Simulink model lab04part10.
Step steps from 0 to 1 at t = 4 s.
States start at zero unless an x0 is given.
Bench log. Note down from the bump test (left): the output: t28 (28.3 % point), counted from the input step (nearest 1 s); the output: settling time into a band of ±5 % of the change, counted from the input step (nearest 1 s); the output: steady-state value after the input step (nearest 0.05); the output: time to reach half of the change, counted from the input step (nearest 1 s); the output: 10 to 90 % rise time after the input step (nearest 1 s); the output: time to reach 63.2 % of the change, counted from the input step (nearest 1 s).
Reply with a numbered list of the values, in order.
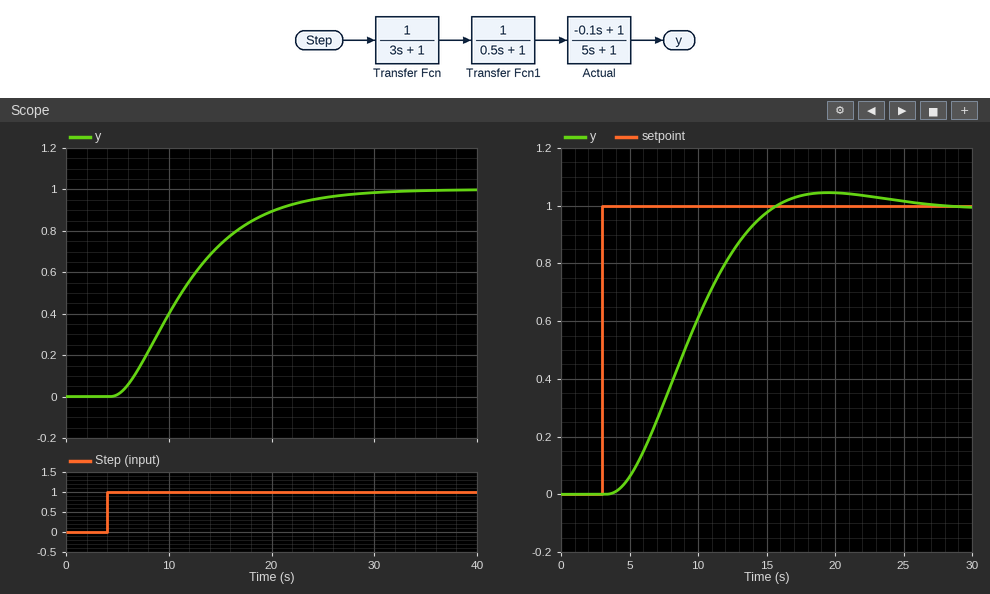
1. 5 s
2. 20 s
3. 1.00
4. 7 s
5. 14 s
6. 9 s
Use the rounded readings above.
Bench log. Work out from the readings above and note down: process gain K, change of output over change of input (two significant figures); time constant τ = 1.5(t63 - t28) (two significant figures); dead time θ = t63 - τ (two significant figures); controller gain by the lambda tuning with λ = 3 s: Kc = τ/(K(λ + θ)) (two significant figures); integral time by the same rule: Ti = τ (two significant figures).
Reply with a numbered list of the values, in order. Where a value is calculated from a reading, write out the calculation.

1. (1 - 0) / 1 = 1.0
2. 1.5 × (9 - 5) = 6.0 s
3. 9 - 6 = 3.0 s
4. 6 / (1 × (3 + 3)) = 1.0
5. 6.0 s
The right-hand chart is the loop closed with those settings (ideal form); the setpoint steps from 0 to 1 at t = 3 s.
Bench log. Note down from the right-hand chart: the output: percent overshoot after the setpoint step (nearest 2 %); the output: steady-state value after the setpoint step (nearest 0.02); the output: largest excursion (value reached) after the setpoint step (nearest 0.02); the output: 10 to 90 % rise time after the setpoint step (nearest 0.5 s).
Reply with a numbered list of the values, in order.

1. 4 %
2. 1.00
3. 1.04
4. 8.0 s
